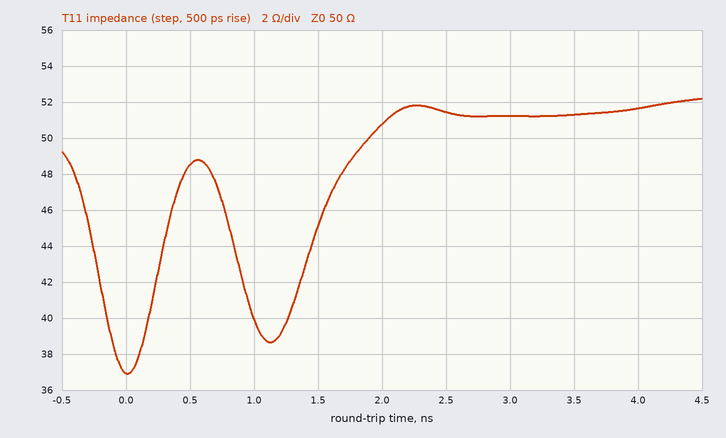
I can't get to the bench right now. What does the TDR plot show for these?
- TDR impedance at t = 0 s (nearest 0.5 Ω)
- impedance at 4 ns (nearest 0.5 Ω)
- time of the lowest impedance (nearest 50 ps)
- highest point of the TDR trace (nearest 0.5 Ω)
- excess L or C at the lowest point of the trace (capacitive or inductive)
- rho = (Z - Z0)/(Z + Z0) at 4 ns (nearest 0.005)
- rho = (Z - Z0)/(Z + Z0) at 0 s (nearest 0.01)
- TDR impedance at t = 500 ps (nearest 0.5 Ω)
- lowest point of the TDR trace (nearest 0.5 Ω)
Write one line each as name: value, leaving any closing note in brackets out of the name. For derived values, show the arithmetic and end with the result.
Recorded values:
TDR impedance at t = 0 s: 37.0 Ω
impedance at 4 ns: 51.5 Ω
time of the lowest impedance: 0 ps
highest point of the TDR trace: 52.0 Ω
excess L or C at the lowest point of the trace: capacitive
rho = (Z - Z0)/(Z + Z0) at 4 ns: (51.5 − 50)/(51.5 + 50) ≈ +0.015
rho = (Z - Z0)/(Z + Z0) at 0 s: (37 − 50)/(37 + 50) ≈ -0.15
TDR impedance at t = 500 ps: 48.5 Ω
lowest point of the TDR trace: 37.0 Ω
